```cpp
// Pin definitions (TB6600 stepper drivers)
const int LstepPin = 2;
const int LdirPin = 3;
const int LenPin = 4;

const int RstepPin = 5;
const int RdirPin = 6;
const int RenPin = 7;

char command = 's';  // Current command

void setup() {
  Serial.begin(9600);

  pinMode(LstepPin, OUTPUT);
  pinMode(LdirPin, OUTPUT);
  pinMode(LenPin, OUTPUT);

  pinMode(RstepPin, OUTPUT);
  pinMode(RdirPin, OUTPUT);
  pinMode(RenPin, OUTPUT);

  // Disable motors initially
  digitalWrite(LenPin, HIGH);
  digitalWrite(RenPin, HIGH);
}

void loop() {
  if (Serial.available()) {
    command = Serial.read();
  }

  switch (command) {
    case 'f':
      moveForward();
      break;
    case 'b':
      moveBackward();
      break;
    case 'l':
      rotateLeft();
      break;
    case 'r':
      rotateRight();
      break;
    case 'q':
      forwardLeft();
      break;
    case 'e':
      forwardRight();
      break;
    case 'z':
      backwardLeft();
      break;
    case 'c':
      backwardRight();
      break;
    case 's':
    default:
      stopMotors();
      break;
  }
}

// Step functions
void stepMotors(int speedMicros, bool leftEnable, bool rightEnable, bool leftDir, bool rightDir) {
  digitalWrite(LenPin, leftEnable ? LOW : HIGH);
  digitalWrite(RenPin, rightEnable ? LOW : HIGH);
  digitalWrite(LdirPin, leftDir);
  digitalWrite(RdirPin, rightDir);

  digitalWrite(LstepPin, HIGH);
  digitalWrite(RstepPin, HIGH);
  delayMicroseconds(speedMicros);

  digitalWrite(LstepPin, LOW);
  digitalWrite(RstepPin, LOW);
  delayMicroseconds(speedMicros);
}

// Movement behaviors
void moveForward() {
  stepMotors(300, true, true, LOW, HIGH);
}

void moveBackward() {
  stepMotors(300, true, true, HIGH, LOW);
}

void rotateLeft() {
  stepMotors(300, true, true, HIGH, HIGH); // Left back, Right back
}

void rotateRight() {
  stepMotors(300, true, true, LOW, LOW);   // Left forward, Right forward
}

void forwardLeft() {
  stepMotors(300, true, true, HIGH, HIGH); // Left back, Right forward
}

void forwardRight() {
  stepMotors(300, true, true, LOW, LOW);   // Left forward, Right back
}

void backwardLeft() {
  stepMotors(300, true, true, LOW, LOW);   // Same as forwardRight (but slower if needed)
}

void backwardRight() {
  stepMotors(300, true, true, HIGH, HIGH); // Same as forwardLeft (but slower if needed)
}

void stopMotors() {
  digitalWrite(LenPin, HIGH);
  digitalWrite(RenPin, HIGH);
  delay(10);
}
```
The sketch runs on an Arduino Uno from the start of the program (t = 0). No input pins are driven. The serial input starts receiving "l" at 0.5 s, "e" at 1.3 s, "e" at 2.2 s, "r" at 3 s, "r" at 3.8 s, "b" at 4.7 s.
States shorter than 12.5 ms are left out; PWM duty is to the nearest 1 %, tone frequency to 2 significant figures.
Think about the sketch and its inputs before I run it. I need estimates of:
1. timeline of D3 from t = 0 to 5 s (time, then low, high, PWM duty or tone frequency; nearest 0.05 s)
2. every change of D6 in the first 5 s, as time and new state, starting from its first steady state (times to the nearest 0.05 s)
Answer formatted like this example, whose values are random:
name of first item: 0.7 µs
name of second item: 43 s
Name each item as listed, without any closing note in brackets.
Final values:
timeline of D3 from t = 0 to 5 s: 0 s low; 0.5 s high; 1.3 s low; 4.7 s high
every change of D6 in the first 5 s, as time and new state, starting from its first steady state: 0 s low; 0.5 s high; 1.3 s low
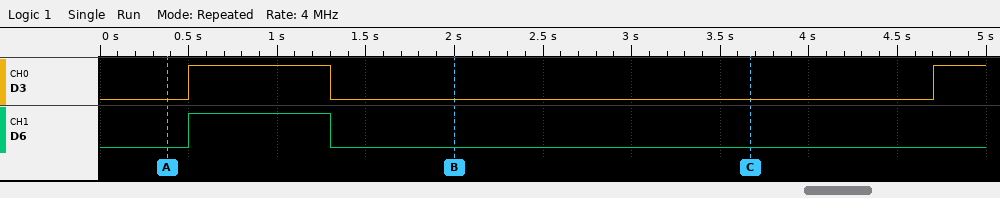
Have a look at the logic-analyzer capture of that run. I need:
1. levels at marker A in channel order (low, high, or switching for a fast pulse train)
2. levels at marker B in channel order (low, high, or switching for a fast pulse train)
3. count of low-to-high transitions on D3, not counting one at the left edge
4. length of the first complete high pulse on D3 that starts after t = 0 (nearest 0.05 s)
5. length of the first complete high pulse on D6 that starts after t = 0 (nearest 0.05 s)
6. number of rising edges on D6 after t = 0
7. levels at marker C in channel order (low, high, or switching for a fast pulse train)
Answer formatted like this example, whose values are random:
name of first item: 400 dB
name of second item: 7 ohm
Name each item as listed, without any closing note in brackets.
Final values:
levels at marker A in channel order: D3 low, D6 low
levels at marker B in channel order: D3 low, D6 low
count of low-to-high transitions on D3, not counting one at the left edge: 2
length of the first complete high pulse on D3 that starts after t = 0: 0.80 s
length of the first complete high pulse on D6 that starts after t = 0: 0.80 s
number of rising edges on D6 after t = 0: 1
levels at marker C in channel order: D3 low, D6 low
